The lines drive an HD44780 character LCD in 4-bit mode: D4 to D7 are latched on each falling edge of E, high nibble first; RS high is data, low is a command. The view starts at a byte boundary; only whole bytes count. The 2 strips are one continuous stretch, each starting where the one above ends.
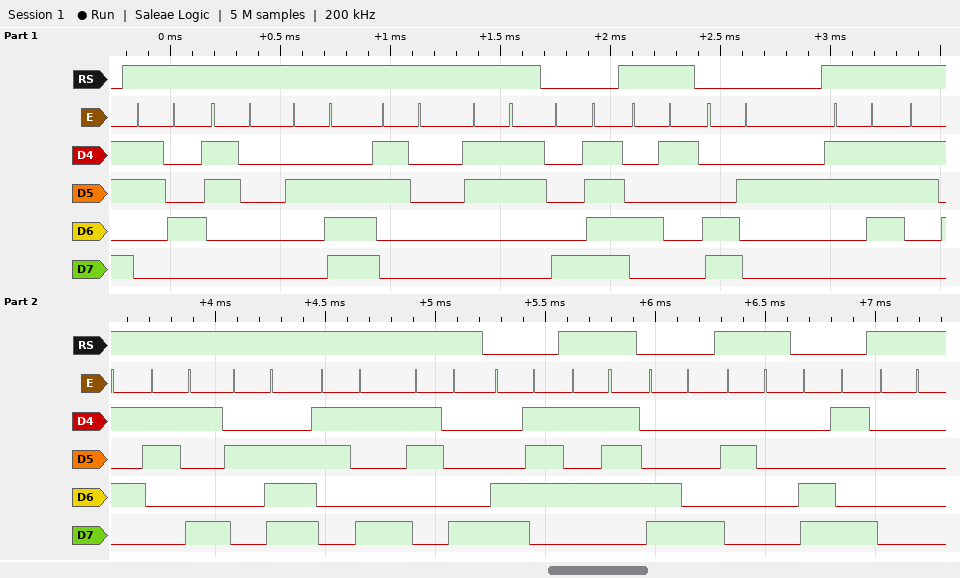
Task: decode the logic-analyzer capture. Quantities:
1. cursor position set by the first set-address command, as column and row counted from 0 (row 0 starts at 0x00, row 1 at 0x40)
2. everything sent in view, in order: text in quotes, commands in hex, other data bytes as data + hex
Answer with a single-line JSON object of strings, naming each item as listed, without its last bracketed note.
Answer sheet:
{"cursor position set by the first set-address command, as column and row counted from 0": "column 15, row 0", "everything sent in view, in order: text in quotes, commands in hex, other data bytes as data + hex": "\"40.03\" 0x8F \"A\" 0xC2 \"759.98\" 0xC7 \"W\" 0xC8 \" \" 0xC9 data 00"}
